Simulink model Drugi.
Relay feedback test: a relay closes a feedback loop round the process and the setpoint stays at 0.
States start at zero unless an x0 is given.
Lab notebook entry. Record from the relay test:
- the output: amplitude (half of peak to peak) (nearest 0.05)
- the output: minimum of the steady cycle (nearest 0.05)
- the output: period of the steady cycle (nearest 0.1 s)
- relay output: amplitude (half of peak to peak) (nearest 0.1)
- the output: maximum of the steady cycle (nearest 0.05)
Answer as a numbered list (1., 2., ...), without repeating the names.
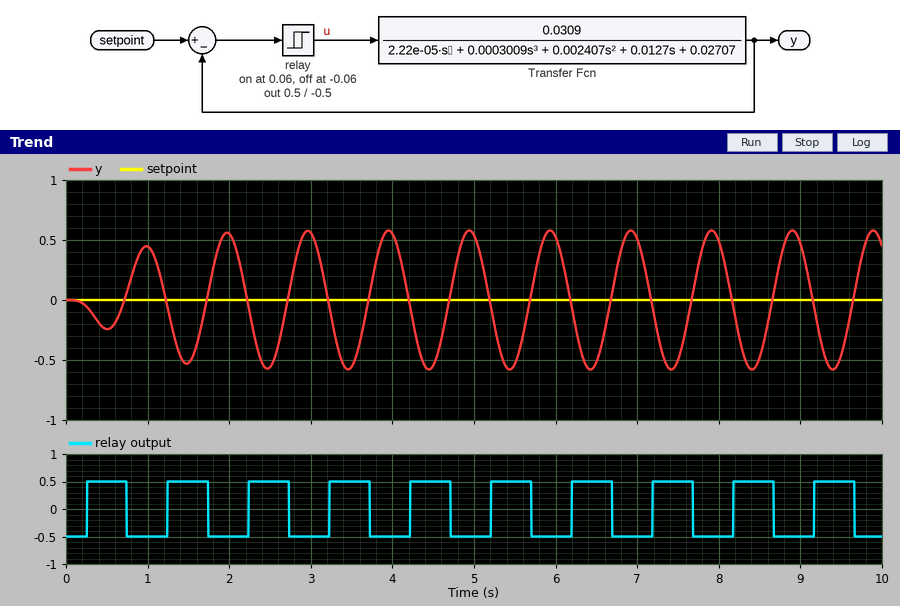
1. 0.60
2. -0.60
3. 1.0 s
4. 0.5
5. 0.60
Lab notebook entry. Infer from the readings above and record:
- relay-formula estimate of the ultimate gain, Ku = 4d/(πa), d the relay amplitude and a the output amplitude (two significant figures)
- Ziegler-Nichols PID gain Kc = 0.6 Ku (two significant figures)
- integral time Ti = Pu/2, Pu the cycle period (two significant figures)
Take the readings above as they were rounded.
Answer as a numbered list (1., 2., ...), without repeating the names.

1. 1.1
2. 0.66
3. 0.50 s
